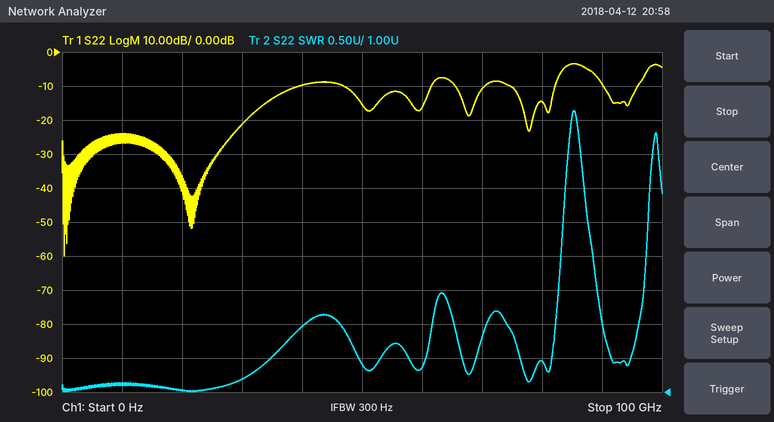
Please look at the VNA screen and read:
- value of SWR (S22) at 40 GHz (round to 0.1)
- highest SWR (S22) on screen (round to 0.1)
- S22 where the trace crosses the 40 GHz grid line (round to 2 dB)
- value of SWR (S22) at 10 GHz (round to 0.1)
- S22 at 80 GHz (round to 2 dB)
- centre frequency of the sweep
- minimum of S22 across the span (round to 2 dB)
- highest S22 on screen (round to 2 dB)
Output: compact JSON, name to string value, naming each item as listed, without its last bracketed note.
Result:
{"value of SWR (S22) at 40 GHz": "2.0", "highest SWR (S22) on screen": "5.1", "S22 where the trace crosses the 40 GHz grid line": "-10 dB", "value of SWR (S22) at 10 GHz": "1.1", "S22 at 80 GHz": "-14 dB", "centre frequency of the sweep": "50 GHz", "minimum of S22 across the span": "-60 dB", "highest S22 on screen": "-4 dB"}
